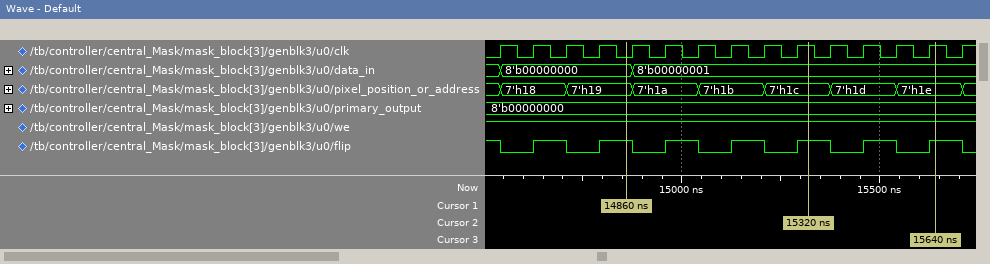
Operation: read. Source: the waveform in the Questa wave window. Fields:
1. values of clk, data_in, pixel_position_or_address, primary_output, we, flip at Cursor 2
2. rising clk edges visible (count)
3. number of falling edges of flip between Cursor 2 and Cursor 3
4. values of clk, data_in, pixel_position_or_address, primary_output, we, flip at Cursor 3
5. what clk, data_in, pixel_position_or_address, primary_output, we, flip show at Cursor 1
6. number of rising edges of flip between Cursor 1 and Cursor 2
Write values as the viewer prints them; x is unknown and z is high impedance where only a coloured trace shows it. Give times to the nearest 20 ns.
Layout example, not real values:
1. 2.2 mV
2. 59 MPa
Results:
1. clk=1, data_in=8'b00000001, pixel_position_or_address=7'h1c, primary_output=8'b00000000, we=1, flip=1
2. 15
3. 2
4. clk=1, data_in=8'b00000001, pixel_position_or_address=7'h1e, primary_output=8'b00000000, we=1, flip=1
5. clk=0, data_in=8'b00000000, pixel_position_or_address=7'h19, primary_output=8'b00000000, we=1, flip=1
6. 3
